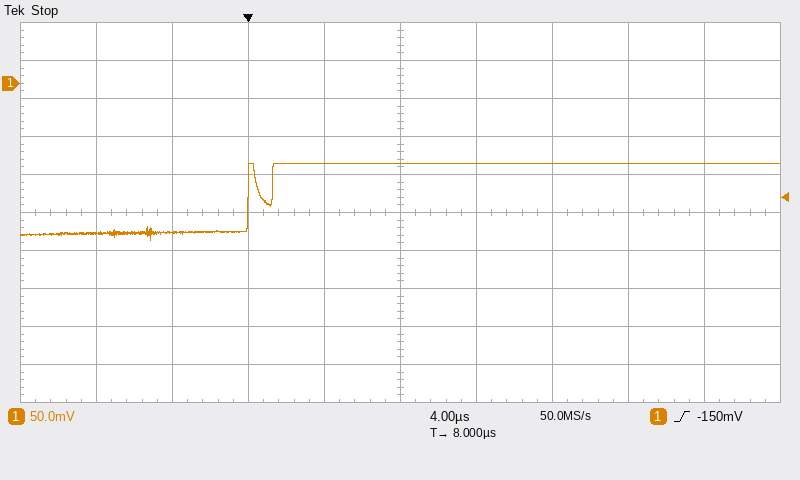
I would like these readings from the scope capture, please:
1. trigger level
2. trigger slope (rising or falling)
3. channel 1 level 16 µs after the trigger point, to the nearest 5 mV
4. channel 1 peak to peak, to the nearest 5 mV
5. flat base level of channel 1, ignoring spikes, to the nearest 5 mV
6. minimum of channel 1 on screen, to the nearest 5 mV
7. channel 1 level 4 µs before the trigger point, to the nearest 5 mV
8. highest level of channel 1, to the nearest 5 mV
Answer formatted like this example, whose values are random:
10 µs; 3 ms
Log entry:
-150 mV; rising; -105 mV; 100 mV; -195 mV; -205 mV; -195 mV; -105 mV
